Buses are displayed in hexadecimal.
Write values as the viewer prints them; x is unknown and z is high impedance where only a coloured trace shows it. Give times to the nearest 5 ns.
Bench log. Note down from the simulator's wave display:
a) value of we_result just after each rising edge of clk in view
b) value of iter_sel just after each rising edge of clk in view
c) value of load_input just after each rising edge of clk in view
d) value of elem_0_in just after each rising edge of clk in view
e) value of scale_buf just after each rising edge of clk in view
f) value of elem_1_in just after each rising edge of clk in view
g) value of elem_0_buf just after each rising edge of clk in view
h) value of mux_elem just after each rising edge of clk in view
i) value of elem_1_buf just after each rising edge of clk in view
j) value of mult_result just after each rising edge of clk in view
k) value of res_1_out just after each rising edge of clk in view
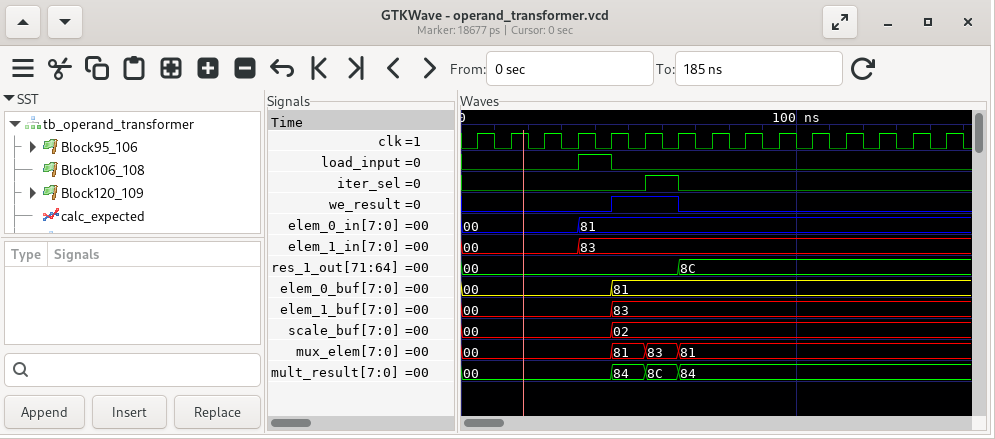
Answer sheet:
0 0 0 0 1 1 0 0 0 0 0 0 0 0 0
0 0 0 0 0 1 0 0 0 0 0 0 0 0 0
0 0 0 1 0 0 0 0 0 0 0 0 0 0 0
00, 00, 00, 81, 81, 81, 81, 81, 81, 81, 81, 81, 81, 81, 81
00, 00, 00, 00, 02, 02, 02, 02, 02, 02, 02, 02, 02, 02, 02
00, 00, 00, 83, 83, 83, 83, 83, 83, 83, 83, 83, 83, 83, 83
00, 00, 00, 00, 81, 81, 81, 81, 81, 81, 81, 81, 81, 81, 81
00, 00, 00, 00, 81, 83, 81, 81, 81, 81, 81, 81, 81, 81, 81
00, 00, 00, 00, 83, 83, 83, 83, 83, 83, 83, 83, 83, 83, 83
00, 00, 00, 00, 84, 8C, 84, 84, 84, 84, 84, 84, 84, 84, 84
00, 00, 00, 00, 00, 00, 8C, 8C, 8C, 8C, 8C, 8C, 8C, 8C, 8C
